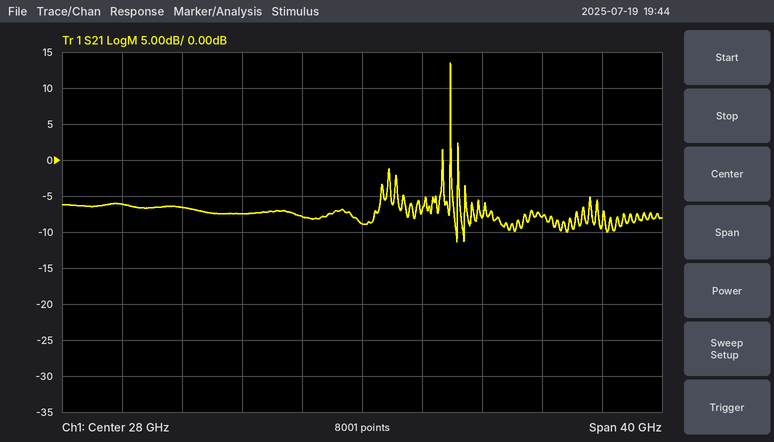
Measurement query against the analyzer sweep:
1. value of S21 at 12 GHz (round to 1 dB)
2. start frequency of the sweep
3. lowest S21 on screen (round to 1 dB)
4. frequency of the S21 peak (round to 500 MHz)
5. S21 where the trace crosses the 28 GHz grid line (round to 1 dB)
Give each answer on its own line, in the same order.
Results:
-6 dB
8 GHz
-11 dB
34.0 GHz
-9 dB
